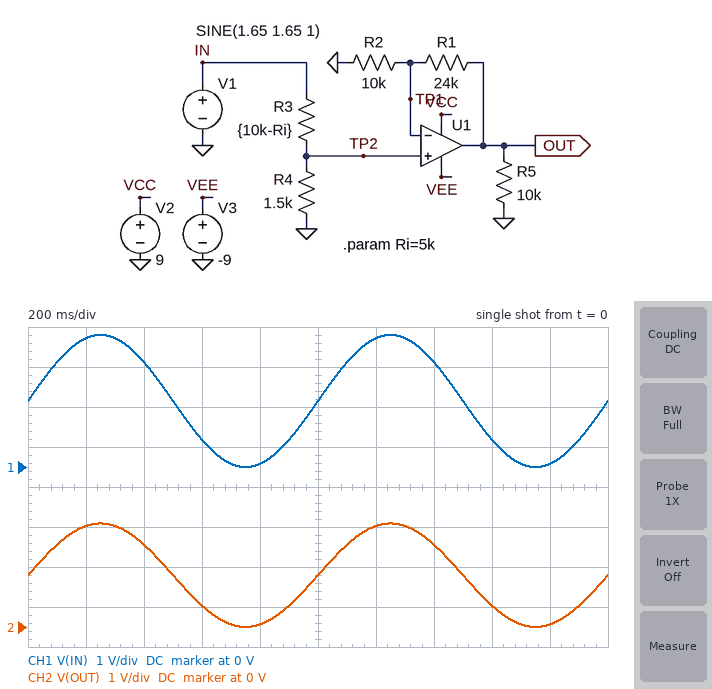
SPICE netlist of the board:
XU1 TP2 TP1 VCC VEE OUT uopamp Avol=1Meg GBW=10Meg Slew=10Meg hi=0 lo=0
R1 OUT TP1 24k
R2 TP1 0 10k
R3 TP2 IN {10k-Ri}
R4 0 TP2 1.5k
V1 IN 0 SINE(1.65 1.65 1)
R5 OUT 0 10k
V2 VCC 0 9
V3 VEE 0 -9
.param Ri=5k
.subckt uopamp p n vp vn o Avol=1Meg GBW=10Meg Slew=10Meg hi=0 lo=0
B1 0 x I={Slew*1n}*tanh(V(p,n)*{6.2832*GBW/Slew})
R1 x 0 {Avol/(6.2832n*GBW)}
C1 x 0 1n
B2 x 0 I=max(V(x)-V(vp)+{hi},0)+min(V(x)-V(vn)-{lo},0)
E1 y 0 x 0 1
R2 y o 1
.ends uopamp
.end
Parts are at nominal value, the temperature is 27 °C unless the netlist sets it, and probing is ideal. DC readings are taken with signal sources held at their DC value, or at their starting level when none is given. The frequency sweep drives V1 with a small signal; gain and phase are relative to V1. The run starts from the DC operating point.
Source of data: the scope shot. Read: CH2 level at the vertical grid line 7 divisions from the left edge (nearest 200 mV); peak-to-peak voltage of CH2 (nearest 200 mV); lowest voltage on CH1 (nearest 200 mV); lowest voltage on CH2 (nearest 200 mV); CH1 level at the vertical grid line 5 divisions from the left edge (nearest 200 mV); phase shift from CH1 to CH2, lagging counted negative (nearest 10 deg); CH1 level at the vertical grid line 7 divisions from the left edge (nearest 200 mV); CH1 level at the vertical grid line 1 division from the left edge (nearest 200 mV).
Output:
2.0 V
2.6 V
0 V
0 V
1.6 V
0 deg
2.6 V
3.2 V
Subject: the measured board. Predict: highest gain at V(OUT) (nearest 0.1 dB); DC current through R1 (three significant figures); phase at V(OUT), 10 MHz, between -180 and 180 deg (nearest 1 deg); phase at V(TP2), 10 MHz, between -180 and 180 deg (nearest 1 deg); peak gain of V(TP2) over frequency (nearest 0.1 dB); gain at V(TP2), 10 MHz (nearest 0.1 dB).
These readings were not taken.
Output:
-2.1 dB
38.1 µA
-74 deg
0 deg
-12.7 dB
-12.7 dB
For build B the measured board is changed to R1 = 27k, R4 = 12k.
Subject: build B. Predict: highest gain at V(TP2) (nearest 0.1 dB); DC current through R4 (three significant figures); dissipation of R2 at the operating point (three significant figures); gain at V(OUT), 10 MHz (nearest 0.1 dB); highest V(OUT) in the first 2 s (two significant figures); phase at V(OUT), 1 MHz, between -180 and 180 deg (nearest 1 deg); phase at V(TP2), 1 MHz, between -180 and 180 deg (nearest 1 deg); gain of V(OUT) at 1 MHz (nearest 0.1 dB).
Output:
-3.0 dB
97.1 µA
136 µW
-3.3 dB
8.6 V
-20 deg
0 deg
7.8 dB
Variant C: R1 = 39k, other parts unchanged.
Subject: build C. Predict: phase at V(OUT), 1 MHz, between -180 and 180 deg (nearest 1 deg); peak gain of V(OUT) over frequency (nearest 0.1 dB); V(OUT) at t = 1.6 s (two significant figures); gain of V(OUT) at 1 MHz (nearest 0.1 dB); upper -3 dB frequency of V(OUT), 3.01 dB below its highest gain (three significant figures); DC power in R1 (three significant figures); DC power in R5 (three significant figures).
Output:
-26 deg
1.1 dB
770 mV
0.1 dB
2.04 MHz
56.5 µW
348 µW
